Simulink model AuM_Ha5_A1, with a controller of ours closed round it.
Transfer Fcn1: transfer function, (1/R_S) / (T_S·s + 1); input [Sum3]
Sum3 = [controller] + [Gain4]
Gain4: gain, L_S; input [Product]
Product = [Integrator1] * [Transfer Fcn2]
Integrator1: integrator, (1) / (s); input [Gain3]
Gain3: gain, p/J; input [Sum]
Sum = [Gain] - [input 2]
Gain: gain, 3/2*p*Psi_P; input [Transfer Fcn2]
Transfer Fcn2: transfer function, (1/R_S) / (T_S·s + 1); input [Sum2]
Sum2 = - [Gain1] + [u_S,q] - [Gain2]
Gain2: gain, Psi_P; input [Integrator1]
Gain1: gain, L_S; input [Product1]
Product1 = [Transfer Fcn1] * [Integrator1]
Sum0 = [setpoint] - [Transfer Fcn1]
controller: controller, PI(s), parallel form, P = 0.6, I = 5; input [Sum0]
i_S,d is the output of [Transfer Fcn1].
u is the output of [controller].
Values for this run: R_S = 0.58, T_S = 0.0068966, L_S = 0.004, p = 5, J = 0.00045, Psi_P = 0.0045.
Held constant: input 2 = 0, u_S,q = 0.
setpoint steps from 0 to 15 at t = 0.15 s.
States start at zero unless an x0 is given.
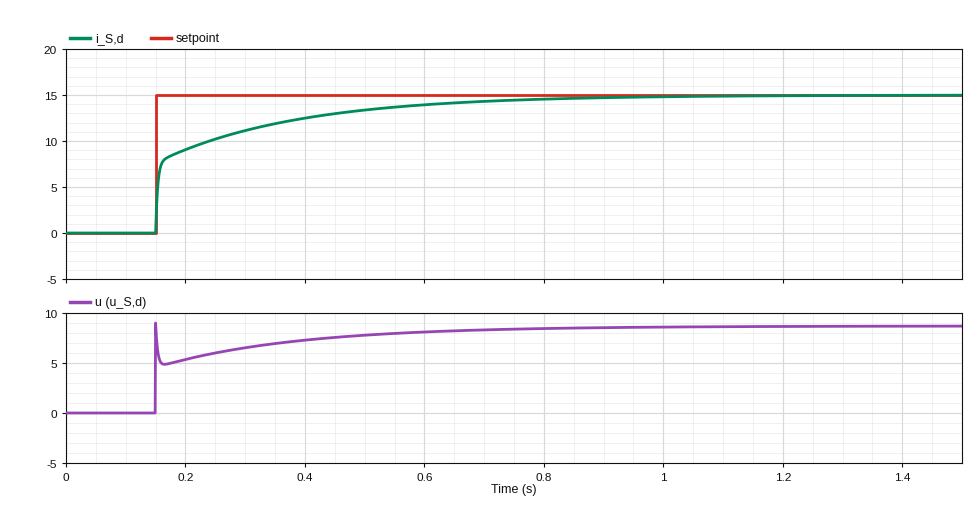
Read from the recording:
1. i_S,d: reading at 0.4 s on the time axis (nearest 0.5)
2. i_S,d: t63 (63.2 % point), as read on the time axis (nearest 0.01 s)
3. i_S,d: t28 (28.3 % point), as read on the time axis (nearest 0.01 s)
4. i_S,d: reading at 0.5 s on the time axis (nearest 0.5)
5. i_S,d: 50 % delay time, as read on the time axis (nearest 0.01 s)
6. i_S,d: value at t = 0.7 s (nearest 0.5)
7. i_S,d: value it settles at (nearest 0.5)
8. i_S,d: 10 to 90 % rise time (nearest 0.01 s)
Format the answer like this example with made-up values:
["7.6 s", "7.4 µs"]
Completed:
["12.5", "0.22 s", "0.15 s", "13.5", "0.16 s", "14.5", "15.0", "0.37 s"]
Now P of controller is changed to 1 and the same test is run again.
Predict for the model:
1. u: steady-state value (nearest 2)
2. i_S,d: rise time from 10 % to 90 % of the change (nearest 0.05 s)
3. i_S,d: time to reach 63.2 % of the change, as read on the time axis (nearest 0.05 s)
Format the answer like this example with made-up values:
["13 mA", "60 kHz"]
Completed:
["8", "0.40 s", "0.15 s"]
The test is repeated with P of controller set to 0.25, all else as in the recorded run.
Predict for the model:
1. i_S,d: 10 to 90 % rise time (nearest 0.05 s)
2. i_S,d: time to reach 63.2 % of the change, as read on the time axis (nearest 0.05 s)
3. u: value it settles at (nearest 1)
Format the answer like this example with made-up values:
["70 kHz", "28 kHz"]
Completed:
["0.30 s", "0.25 s", "9"]
